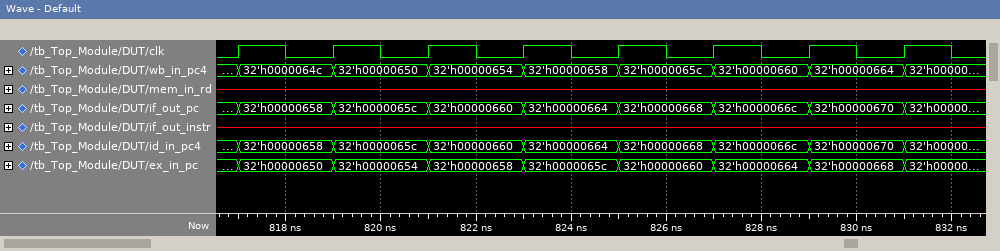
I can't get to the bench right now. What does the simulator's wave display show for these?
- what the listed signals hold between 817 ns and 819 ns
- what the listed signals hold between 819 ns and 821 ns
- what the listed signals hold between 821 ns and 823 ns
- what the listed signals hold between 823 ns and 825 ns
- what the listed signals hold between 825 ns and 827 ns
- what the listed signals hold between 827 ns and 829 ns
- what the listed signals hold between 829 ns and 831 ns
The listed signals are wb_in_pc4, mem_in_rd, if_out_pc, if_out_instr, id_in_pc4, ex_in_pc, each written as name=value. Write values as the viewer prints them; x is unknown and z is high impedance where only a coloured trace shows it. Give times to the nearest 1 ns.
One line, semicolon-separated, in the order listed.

wb_in_pc4=32'h0000064c, mem_in_rd=x, if_out_pc=32'h00000658, if_out_instr=x, id_in_pc4=32'h00000658, ex_in_pc=32'h00000650; wb_in_pc4=32'h00000650, mem_in_rd=x, if_out_pc=32'h0000065c, if_out_instr=x, id_in_pc4=32'h0000065c, ex_in_pc=32'h00000654; wb_in_pc4=32'h00000654, mem_in_rd=x, if_out_pc=32'h00000660, if_out_instr=x, id_in_pc4=32'h00000660, ex_in_pc=32'h00000658; wb_in_pc4=32'h00000658, mem_in_rd=x, if_out_pc=32'h00000664, if_out_instr=x, id_in_pc4=32'h00000664, ex_in_pc=32'h0000065c; wb_in_pc4=32'h0000065c, mem_in_rd=x, if_out_pc=32'h00000668, if_out_instr=x, id_in_pc4=32'h00000668, ex_in_pc=32'h00000660; wb_in_pc4=32'h00000660, mem_in_rd=x, if_out_pc=32'h0000066c, if_out_instr=x, id_in_pc4=32'h0000066c, ex_in_pc=32'h00000664; wb_in_pc4=32'h00000664, mem_in_rd=x, if_out_pc=32'h00000670, if_out_instr=x, id_in_pc4=32'h00000670, ex_in_pc=32'h00000668
